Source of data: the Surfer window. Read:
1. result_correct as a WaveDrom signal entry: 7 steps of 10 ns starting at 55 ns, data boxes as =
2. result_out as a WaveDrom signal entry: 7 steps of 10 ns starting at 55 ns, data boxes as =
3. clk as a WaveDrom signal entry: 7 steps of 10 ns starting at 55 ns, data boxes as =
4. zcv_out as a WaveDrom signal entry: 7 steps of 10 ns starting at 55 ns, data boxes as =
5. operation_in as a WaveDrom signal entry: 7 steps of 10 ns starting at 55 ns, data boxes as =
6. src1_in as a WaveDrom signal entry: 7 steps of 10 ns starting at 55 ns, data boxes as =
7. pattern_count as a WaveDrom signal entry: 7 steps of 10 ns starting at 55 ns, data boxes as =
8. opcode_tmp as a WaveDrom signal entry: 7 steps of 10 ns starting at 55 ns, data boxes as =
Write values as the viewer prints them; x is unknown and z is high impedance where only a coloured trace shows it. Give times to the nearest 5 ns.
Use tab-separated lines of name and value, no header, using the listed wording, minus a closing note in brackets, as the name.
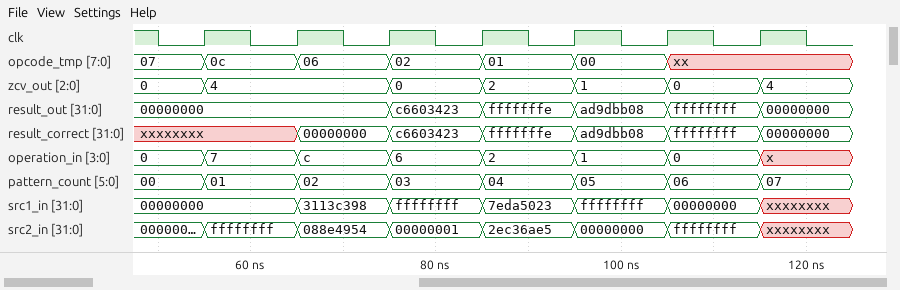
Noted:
result_correct as a WaveDrom signal entry: 7 steps of 10 ns starting at 55 ns, data boxes as =	{name: 'result_correct', wave: 'x======', data: '00000000 c6603423 fffffffe ad9dbb08 ffffffff 00000000'}
result_out as a WaveDrom signal entry: 7 steps of 10 ns starting at 55 ns, data boxes as =	{name: 'result_out', wave: '=.=====', data: '00000000 c6603423 fffffffe ad9dbb08 ffffffff 00000000'}
clk as a WaveDrom signal entry: 7 steps of 10 ns starting at 55 ns, data boxes as =	{name: 'clk', wave: 'p......'}
zcv_out as a WaveDrom signal entry: 7 steps of 10 ns starting at 55 ns, data boxes as =	{name: 'zcv_out', wave: '=.=====', data: '4 0 2 1 0 4'}
operation_in as a WaveDrom signal entry: 7 steps of 10 ns starting at 55 ns, data boxes as =	{name: 'operation_in', wave: '======x', data: '7 c 6 2 1 0'}
src1_in as a WaveDrom signal entry: 7 steps of 10 ns starting at 55 ns, data boxes as =	{name: 'src1_in', wave: '======x', data: '00000000 3113c398 ffffffff 7eda5023 ffffffff 00000000'}
pattern_count as a WaveDrom signal entry: 7 steps of 10 ns starting at 55 ns, data boxes as =	{name: 'pattern_count', wave: '=======', data: '01 02 03 04 05 06 07'}
opcode_tmp as a WaveDrom signal entry: 7 steps of 10 ns starting at 55 ns, data boxes as =	{name: 'opcode_tmp', wave: '=====x.', data: '0c 06 02 01 00'}
